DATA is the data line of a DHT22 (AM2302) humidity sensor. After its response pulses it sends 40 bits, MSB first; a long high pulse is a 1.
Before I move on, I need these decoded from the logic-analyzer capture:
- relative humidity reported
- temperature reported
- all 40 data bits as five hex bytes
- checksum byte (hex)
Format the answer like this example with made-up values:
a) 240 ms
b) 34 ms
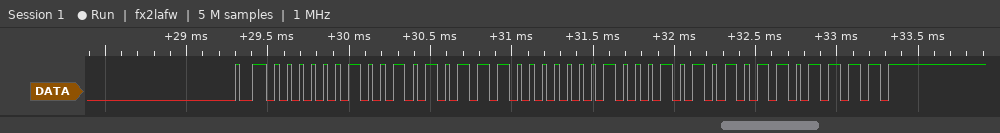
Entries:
a) 59.9 %
b) 27.7 °C
c) 02 57 01 15 6F
d) 0x6F
